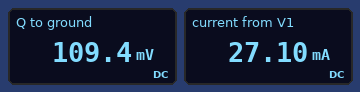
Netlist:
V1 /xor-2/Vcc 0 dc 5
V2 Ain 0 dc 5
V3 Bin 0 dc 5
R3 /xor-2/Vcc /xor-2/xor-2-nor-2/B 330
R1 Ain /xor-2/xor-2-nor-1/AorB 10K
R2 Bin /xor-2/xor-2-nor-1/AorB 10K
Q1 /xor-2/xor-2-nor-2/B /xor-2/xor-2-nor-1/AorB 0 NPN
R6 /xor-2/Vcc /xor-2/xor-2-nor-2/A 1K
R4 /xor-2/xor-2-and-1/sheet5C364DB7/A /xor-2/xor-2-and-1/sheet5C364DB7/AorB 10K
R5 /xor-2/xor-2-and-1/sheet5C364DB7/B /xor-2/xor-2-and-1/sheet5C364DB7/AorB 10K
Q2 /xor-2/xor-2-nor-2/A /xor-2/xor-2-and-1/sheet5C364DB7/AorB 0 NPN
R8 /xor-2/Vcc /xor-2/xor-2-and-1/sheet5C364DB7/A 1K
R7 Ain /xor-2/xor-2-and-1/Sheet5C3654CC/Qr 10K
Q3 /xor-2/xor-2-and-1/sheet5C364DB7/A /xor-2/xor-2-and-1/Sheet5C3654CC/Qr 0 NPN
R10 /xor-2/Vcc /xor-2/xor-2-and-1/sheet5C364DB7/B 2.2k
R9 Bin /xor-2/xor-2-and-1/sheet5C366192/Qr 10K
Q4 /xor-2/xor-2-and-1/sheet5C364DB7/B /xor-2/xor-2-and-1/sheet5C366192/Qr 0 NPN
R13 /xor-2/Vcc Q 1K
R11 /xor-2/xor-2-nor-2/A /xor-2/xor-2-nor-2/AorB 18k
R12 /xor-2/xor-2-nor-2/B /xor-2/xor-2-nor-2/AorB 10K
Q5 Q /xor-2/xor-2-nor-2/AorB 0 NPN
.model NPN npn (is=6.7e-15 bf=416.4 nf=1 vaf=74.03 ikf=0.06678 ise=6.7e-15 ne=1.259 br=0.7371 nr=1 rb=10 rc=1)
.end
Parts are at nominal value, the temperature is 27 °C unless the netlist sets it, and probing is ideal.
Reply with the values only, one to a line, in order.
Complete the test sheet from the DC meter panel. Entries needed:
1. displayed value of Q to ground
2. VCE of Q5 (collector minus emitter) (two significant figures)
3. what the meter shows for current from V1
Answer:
109.4 mV
110 mV
27.10 mA
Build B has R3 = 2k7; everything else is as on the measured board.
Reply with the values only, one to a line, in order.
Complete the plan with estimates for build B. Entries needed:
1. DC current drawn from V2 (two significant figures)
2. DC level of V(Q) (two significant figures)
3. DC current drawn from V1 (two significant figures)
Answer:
860 µA
110 mV
14 mA
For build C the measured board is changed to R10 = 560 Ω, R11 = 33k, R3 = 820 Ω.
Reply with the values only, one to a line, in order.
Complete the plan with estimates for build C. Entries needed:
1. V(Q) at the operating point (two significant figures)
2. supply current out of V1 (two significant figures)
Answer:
150 mV
25 mA
